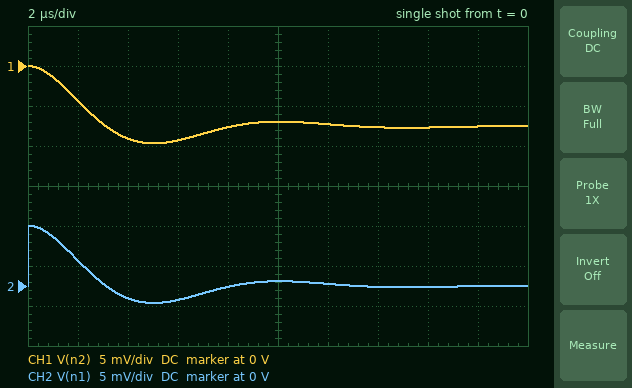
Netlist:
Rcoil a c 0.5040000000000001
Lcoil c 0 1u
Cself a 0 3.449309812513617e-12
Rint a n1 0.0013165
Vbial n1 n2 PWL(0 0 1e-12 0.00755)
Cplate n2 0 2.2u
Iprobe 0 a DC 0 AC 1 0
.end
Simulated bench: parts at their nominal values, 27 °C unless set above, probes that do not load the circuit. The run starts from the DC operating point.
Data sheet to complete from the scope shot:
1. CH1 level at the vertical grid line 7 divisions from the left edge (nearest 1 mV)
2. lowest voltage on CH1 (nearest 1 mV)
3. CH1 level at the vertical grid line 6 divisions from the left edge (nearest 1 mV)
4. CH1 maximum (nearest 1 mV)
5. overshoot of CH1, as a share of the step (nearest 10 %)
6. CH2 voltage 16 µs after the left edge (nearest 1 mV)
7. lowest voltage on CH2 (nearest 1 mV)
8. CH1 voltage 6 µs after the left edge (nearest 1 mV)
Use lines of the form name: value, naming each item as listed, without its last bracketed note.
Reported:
CH1 level at the vertical grid line 7 divisions from the left edge: -8 mV
lowest voltage on CH1: -10 mV
CH1 level at the vertical grid line 6 divisions from the left edge: -7 mV
CH1 maximum: 0 V
overshoot of CH1, as a share of the step: 30 %
CH2 voltage 16 µs after the left edge: 0 V
lowest voltage on CH2: -2 mV
CH1 voltage 6 µs after the left edge: -9 mV
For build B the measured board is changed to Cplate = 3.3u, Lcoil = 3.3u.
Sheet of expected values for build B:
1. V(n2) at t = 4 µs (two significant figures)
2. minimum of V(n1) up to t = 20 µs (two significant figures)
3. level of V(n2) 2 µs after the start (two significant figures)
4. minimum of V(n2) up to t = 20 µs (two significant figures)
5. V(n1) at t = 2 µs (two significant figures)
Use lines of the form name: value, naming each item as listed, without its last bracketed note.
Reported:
V(n2) at t = 4 µs: -4.1 mV
minimum of V(n1) up to t = 20 µs: -3.3 mV
level of V(n2) 2 µs after the start: -1.2 mV
minimum of V(n2) up to t = 20 µs: -11 mV
V(n1) at t = 2 µs: 6.3 mV
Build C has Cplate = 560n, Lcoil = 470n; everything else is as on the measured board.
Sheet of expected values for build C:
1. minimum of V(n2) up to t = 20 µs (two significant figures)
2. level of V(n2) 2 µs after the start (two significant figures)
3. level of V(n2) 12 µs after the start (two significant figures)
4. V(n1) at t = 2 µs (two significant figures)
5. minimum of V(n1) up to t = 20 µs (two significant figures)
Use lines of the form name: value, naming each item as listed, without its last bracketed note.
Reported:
minimum of V(n2) up to t = 20 µs: -11 mV
level of V(n2) 2 µs after the start: -10 mV
level of V(n2) 12 µs after the start: -7.6 mV
V(n1) at t = 2 µs: -2.5 mV
minimum of V(n1) up to t = 20 µs: -3.1 mV
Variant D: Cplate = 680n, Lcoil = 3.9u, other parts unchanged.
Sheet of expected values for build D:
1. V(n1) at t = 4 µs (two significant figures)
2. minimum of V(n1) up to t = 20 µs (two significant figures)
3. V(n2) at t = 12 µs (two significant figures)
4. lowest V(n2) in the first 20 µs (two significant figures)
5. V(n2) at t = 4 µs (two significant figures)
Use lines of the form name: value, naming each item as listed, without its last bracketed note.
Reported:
V(n1) at t = 4 µs: -4.1 mV
minimum of V(n1) up to t = 20 µs: -5.4 mV
V(n2) at t = 12 µs: -5.5 mV
lowest V(n2) in the first 20 µs: -13 mV
V(n2) at t = 4 µs: -12 mV
